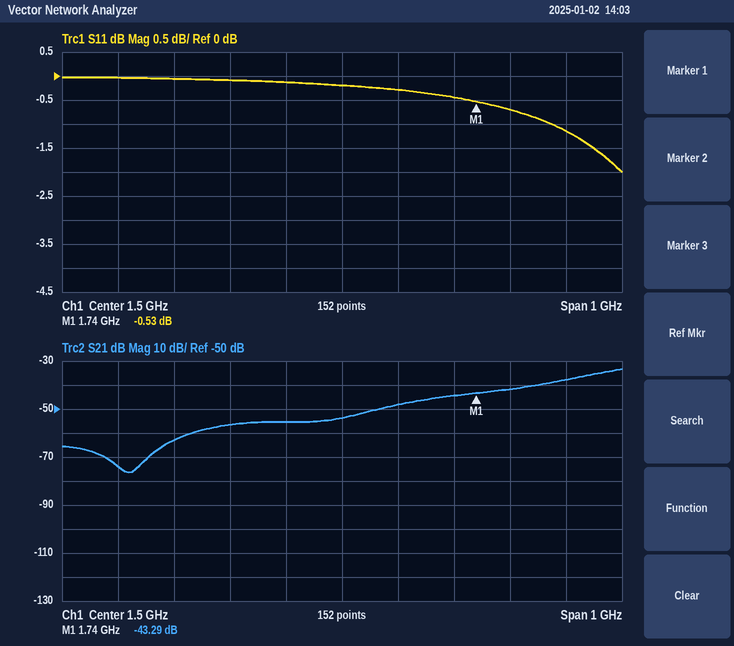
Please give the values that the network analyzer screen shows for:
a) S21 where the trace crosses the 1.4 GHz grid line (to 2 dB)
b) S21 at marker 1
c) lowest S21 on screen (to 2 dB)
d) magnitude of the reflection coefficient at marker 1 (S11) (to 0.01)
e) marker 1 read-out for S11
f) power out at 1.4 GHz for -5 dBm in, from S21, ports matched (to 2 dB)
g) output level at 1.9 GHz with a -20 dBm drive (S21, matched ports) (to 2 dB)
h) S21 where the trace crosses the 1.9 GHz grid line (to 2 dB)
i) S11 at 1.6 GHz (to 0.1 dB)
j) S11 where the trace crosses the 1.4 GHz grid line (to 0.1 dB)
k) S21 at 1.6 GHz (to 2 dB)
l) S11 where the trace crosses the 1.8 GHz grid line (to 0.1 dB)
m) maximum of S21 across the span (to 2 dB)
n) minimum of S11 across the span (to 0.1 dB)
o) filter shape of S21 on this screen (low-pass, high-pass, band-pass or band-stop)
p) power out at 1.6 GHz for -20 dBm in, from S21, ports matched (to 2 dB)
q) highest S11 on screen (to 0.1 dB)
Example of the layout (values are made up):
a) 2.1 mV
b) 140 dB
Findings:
a) -56 dB
b) -43.29 dB
c) -76 dB
d) 0.94
e) -0.53 dB
f) -60 dBm
g) -58 dBm
h) -38 dB
i) -0.3 dB
j) -0.1 dB
k) -48 dB
l) -0.7 dB
m) -34 dB
n) -2.0 dB
o) high-pass
p) -68 dBm
q) 0.0 dB
